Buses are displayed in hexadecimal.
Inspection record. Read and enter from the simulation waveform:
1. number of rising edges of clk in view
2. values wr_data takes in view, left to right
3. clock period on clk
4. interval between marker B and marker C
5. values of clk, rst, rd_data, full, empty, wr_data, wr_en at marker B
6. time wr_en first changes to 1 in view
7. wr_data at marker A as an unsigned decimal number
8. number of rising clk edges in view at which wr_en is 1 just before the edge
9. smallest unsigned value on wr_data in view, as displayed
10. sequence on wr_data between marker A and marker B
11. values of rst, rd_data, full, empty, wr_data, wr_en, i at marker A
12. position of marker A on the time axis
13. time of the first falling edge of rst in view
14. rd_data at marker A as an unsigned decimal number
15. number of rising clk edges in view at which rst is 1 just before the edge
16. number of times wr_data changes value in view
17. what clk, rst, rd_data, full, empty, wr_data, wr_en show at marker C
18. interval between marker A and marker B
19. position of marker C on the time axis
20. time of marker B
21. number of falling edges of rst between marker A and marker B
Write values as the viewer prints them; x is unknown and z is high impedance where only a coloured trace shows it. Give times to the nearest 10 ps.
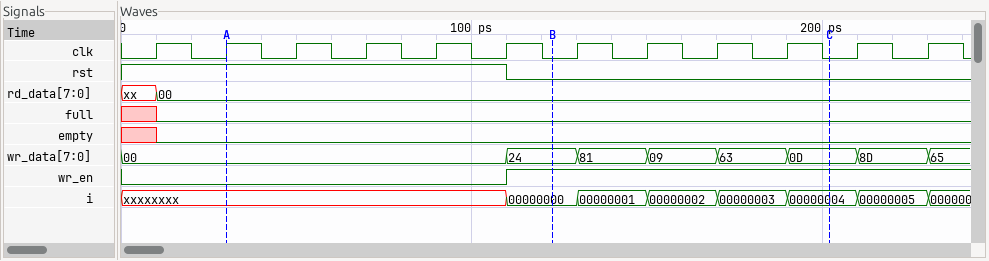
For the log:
12
00, 24, 81, 09, 63, 0D, 8D, 65
20 ps
80 ps
clk=0, rst=0, rd_data=00, full=0, empty=0, wr_data=24, wr_en=1
110 ps
0
6
00
00, 24
rst=1, rd_data=00, full=0, empty=0, wr_data=00, wr_en=0, i=xxxxxxxx
30 ps
110 ps
0
6
7
clk=0, rst=0, rd_data=00, full=0, empty=0, wr_data=0D, wr_en=1
90 ps
200 ps
120 ps
1
